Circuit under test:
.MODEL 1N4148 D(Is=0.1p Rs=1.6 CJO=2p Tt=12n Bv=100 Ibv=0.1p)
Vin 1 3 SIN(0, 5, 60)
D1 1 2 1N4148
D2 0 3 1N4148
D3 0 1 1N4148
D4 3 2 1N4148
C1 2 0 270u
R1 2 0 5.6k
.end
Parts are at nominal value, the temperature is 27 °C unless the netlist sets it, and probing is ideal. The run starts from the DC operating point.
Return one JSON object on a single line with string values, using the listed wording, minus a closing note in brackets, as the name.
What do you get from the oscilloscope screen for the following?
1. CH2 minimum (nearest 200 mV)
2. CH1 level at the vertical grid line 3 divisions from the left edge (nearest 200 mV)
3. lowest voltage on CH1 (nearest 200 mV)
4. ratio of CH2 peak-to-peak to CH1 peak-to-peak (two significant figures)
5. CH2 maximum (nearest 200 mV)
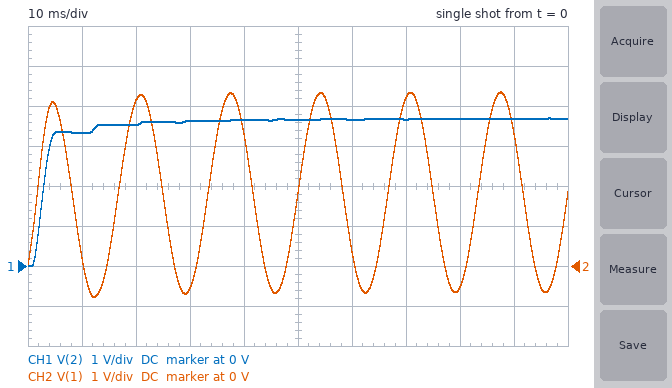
{"CH2 minimum": "-800 mV", "CH1 level at the vertical grid line 3 divisions from the left edge": "3.6 V", "lowest voltage on CH1": "0 V", "ratio of CH2 peak-to-peak to CH1 peak-to-peak": "1.4", "CH2 maximum": "4.4 V"}
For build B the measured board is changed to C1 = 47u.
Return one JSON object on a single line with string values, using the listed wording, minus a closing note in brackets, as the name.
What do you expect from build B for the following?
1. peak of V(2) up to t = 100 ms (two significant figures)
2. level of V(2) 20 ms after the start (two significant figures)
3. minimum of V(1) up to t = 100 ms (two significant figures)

{"peak of V(2) up to t = 100 ms": "3.7 V", "level of V(2) 20 ms after the start": "3.6 V", "minimum of V(1) up to t = 100 ms": "-660 mV"}
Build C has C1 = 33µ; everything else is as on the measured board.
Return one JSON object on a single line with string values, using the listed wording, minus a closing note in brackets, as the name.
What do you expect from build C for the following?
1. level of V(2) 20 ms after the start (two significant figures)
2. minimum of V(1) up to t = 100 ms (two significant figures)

{"level of V(2) 20 ms after the start": "3.6 V", "minimum of V(1) up to t = 100 ms": "-660 mV"}
